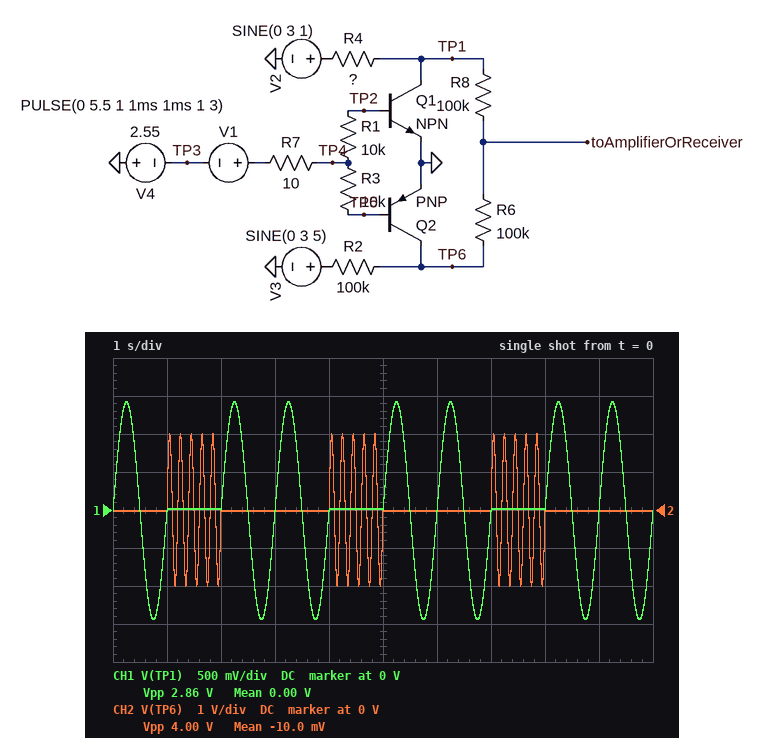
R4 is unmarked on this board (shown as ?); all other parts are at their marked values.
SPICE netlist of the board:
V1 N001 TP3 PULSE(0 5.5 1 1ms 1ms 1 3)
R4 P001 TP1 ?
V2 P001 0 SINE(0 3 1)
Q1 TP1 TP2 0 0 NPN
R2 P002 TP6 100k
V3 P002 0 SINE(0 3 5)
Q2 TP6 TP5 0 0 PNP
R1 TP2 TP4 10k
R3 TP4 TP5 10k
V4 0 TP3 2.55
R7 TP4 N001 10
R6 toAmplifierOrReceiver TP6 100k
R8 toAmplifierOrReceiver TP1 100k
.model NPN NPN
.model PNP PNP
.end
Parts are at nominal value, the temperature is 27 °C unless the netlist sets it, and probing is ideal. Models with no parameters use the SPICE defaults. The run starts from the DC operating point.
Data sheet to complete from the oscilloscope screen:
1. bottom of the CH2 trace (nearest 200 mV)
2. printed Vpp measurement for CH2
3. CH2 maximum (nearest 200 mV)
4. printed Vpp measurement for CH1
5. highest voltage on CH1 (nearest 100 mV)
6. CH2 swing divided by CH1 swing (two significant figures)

-2.0 V
4.00 V
2.0 V
2.86 V
1.4 V
1.4
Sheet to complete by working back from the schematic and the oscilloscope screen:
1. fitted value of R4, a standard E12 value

220 kΩ
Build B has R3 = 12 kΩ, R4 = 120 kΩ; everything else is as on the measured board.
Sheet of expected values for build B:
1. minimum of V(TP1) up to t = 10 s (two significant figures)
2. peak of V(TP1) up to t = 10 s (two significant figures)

-1.9 V
1.9 V
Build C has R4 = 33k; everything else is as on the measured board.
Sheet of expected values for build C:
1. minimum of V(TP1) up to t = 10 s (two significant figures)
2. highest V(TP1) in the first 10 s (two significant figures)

-2.6 V
2.6 V
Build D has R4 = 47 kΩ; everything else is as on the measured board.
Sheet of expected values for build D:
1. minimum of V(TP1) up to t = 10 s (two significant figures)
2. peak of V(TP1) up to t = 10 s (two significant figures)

-2.4 V
2.4 V
